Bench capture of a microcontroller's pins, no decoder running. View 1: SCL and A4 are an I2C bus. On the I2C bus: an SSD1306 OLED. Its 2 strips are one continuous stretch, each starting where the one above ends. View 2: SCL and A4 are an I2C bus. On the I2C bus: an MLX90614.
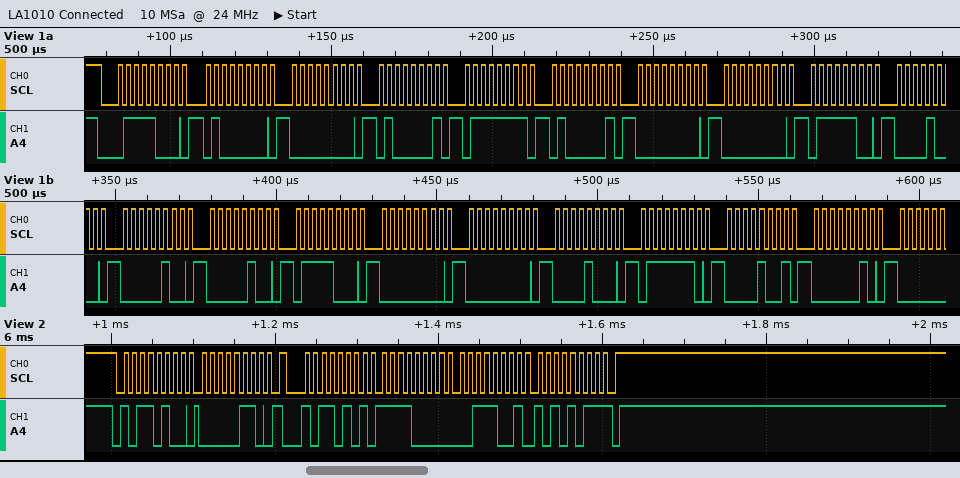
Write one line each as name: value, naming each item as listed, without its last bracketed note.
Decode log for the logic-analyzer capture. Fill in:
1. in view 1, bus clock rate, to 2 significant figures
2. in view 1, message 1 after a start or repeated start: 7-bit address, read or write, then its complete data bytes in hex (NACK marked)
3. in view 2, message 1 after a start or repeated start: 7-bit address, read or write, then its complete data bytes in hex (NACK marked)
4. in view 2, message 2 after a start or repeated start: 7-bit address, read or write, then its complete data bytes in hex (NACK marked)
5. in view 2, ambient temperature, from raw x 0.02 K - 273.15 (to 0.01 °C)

in view 1, bus clock rate, to 2 significant figures: 400 kHz
in view 1, message 1 after a start or repeated start: 7-bit address, read or write, then its complete data bytes in hex: 0x3C write: 40 00 41 7F 41 00 00 7C 08 04 04 78 00 00 08 7E 09 02
in view 2, message 1 after a start or repeated start: 7-bit address, read or write, then its complete data bytes in hex: 0x5A write: 06
in view 2, message 2 after a start or repeated start: 7-bit address, read or write, then its complete data bytes in hex: 0x5A read: F0 39 AB NACK
in view 2, ambient temperature, from raw x 0.02 K - 273.15: 23.49 °C
